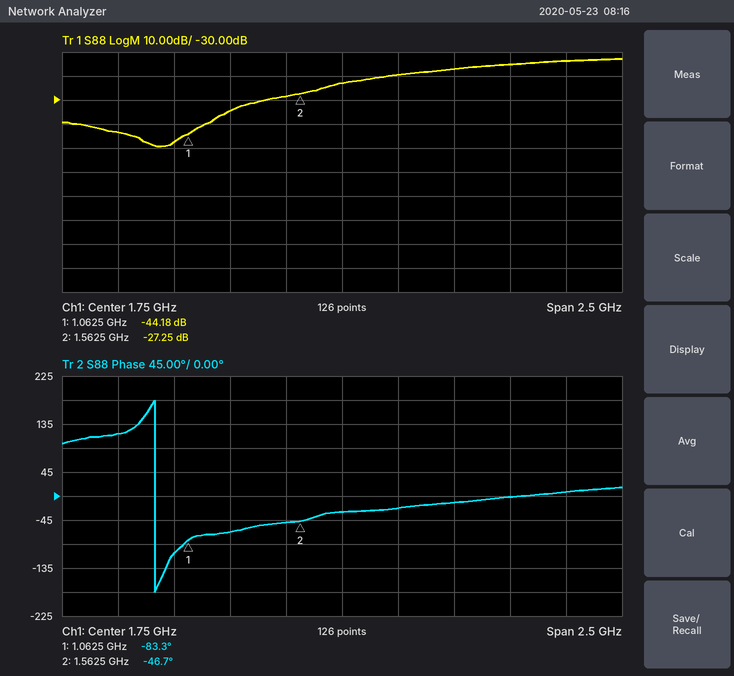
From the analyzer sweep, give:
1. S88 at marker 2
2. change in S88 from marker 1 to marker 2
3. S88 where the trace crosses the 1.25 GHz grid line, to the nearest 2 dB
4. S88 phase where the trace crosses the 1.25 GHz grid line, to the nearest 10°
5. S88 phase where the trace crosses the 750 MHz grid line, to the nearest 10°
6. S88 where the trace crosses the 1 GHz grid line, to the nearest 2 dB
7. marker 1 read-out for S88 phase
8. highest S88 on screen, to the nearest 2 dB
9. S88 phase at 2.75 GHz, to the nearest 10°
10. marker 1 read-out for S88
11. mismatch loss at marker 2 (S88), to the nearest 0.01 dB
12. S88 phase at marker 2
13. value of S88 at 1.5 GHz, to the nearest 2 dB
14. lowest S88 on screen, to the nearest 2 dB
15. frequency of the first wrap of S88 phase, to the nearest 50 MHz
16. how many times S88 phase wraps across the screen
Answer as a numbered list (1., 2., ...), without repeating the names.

1. -27.25 dB
2. 16.93 dB
3. -34 dB
4. -70°
5. 120°
6. -48 dB
7. -83.3°
8. -12 dB
9. 10°
10. -44.18 dB
11. 0.01 dB
12. -46.7°
13. -28 dB
14. -50 dB
15. 900 MHz
16. 1
